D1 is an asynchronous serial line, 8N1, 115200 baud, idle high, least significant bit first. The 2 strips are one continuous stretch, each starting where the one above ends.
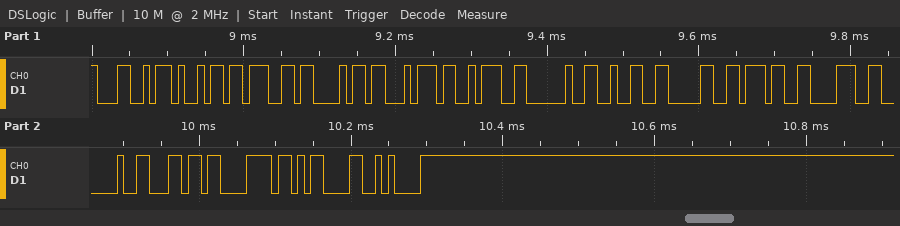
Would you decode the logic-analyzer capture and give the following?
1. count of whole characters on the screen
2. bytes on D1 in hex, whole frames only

16
0x4C 0x69 0x67 0x68 0x74 0x3A 0x20 0x32 0x30 0x37 0x38 0x20 0x6C 0x78 0x0D 0x0A
